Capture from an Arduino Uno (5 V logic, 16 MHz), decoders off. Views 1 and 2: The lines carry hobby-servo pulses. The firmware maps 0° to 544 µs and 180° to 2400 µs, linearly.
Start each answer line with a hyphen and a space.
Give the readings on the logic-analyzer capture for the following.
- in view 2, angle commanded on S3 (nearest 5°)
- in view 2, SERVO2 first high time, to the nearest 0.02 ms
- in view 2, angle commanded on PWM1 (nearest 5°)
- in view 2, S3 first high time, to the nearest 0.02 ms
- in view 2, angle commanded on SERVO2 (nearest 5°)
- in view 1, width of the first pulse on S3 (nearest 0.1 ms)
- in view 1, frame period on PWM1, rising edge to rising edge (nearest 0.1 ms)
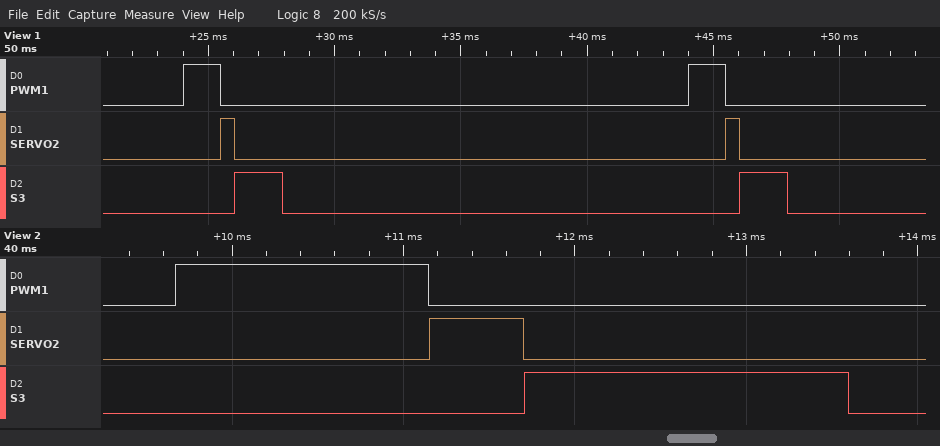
- 130°
- 0.54 ms
- 90°
- 1.88 ms
- 0°
- 1.9 ms
- 20.0 ms
